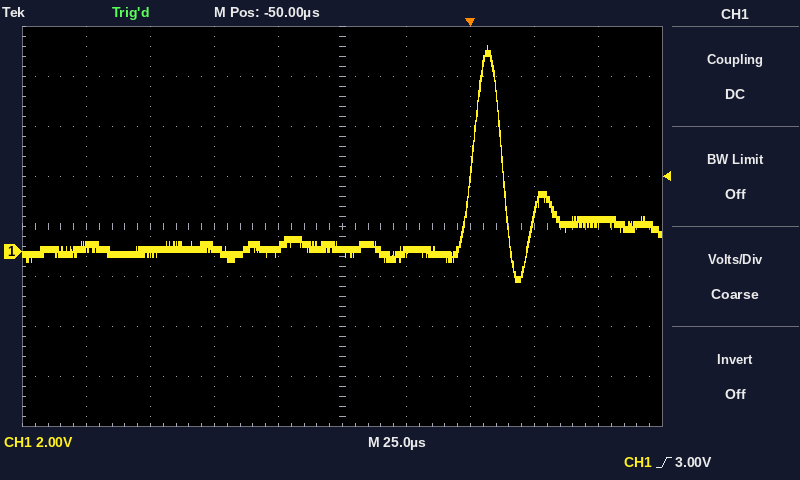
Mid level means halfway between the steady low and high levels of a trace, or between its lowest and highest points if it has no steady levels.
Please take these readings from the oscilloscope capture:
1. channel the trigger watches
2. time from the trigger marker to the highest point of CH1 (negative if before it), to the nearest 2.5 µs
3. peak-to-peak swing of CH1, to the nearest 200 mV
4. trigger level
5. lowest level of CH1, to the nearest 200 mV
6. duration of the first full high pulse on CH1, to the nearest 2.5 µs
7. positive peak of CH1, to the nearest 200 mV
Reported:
CH1
+7.5 µs
9.4 V
3.00 V
-1.2 V
12.5 µs
8.2 V
